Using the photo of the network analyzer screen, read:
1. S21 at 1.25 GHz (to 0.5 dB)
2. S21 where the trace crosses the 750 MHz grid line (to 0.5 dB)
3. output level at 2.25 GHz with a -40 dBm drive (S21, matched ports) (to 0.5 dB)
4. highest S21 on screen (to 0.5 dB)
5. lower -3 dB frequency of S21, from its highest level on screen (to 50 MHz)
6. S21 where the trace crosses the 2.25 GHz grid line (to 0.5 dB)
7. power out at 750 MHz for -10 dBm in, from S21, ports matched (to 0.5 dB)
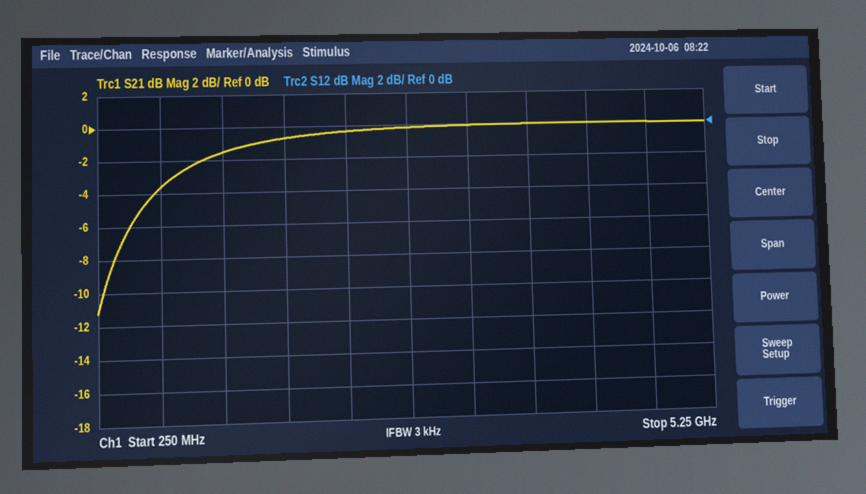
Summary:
-1.5 dB
-3.5 dB
-40.5 dBm
0.0 dB
850 MHz
-0.5 dB
-13.5 dBm
